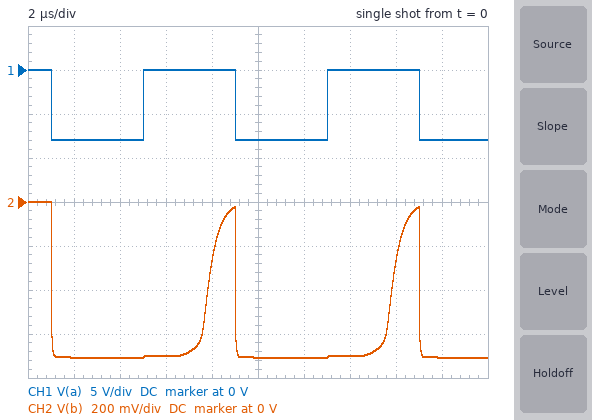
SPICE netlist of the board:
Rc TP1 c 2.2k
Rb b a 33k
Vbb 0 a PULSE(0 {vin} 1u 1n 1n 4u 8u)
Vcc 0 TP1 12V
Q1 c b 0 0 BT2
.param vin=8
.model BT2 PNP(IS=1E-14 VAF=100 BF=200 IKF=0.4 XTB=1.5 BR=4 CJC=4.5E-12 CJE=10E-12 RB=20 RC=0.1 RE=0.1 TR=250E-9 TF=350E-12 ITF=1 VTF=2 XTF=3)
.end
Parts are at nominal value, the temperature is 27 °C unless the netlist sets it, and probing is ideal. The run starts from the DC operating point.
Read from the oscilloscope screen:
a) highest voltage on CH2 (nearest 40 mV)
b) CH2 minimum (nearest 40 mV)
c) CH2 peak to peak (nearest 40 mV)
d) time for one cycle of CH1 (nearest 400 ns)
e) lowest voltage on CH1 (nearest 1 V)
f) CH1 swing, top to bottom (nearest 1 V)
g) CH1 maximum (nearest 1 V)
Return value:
0 V
-720 mV
720 mV
8.0 µs
-8 V
8 V
0 V
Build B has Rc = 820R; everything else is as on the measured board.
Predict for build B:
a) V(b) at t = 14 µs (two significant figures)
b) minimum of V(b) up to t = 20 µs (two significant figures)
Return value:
-720 mV
-730 mV
